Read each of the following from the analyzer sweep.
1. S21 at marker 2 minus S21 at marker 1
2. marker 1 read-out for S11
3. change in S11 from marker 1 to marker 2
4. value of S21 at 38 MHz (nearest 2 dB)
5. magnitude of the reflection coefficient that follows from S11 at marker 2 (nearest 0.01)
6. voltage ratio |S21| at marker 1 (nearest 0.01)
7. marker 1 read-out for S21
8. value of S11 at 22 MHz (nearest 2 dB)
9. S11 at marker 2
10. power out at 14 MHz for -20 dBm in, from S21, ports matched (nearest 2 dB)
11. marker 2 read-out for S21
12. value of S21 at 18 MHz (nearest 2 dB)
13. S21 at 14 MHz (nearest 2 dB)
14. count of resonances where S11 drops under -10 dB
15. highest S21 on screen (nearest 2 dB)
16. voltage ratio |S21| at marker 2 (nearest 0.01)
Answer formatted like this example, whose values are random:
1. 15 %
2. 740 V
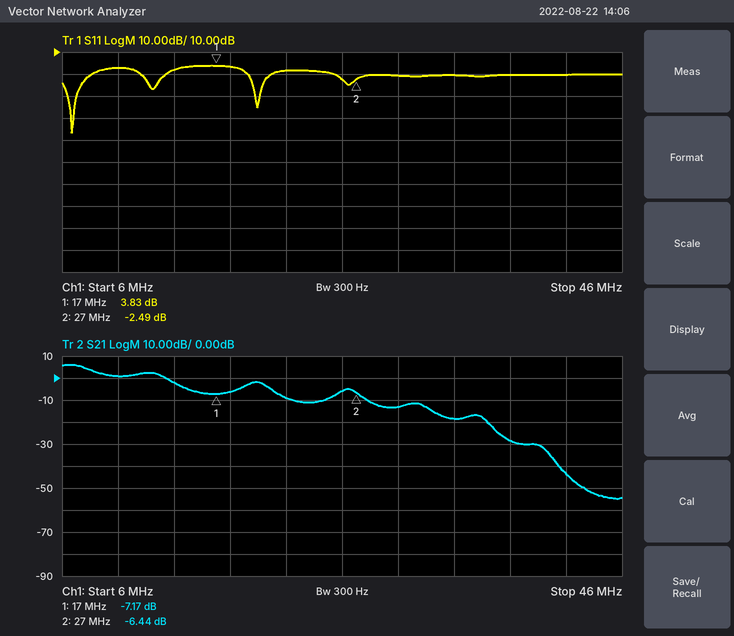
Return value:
1. 0.73 dB
2. 3.83 dB
3. -6.32 dB
4. -28 dB
5. 0.75
6. 0.44
7. -7.17 dB
8. 2 dB
9. -2.49 dB
10. -22 dBm
11. -6.44 dB
12. -6 dB
13. -2 dB
14. 2
15. 6 dB
16. 0.48
